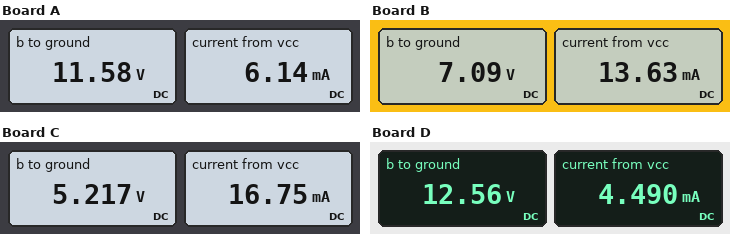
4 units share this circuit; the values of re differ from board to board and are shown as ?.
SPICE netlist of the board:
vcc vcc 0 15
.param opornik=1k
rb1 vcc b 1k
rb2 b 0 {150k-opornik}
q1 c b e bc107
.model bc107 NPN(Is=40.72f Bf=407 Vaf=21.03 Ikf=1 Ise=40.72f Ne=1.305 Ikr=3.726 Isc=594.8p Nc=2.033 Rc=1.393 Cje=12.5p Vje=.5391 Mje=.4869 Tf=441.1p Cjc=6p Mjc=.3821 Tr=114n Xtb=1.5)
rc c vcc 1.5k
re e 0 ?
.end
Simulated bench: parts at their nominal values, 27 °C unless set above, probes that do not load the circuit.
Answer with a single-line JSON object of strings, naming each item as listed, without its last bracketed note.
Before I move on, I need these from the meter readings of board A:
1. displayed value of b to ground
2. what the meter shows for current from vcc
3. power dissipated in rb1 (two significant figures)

{"displayed value of b to ground": "11.58 V", "what the meter shows for current from vcc": "6.14 mA", "power dissipated in rb1": "12 mW"}
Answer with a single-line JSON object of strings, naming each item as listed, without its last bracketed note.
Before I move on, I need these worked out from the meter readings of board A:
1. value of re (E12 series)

{"value of re": "1.8 kΩ"}
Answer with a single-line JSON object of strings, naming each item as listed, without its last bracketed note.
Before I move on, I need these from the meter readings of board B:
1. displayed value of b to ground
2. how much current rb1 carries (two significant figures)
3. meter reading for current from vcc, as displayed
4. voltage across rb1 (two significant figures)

{"displayed value of b to ground": "7.09 V", "how much current rb1 carries": "7.9 mA", "meter reading for current from vcc, as displayed": "13.63 mA", "voltage across rb1": "7.9 V"}
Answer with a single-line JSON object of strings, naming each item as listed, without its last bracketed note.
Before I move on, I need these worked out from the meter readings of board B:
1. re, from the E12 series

{"re, from the E12 series": "470 Ω"}
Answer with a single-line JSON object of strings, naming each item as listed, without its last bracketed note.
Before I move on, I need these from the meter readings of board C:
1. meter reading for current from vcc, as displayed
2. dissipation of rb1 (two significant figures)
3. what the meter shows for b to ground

{"meter reading for current from vcc, as displayed": "16.75 mA", "dissipation of rb1": "96 mW", "what the meter shows for b to ground": "5.217 V"}
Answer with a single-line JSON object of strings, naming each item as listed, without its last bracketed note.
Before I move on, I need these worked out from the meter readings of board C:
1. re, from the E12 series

{"re, from the E12 series": "270 Ω"}
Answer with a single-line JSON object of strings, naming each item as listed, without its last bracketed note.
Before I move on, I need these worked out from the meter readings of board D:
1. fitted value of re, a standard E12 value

{"fitted value of re, a standard E12 value": "2.7 kΩ"}
